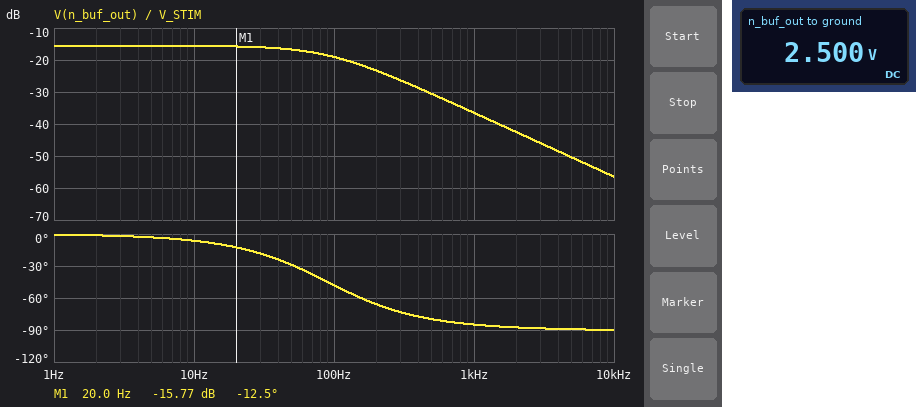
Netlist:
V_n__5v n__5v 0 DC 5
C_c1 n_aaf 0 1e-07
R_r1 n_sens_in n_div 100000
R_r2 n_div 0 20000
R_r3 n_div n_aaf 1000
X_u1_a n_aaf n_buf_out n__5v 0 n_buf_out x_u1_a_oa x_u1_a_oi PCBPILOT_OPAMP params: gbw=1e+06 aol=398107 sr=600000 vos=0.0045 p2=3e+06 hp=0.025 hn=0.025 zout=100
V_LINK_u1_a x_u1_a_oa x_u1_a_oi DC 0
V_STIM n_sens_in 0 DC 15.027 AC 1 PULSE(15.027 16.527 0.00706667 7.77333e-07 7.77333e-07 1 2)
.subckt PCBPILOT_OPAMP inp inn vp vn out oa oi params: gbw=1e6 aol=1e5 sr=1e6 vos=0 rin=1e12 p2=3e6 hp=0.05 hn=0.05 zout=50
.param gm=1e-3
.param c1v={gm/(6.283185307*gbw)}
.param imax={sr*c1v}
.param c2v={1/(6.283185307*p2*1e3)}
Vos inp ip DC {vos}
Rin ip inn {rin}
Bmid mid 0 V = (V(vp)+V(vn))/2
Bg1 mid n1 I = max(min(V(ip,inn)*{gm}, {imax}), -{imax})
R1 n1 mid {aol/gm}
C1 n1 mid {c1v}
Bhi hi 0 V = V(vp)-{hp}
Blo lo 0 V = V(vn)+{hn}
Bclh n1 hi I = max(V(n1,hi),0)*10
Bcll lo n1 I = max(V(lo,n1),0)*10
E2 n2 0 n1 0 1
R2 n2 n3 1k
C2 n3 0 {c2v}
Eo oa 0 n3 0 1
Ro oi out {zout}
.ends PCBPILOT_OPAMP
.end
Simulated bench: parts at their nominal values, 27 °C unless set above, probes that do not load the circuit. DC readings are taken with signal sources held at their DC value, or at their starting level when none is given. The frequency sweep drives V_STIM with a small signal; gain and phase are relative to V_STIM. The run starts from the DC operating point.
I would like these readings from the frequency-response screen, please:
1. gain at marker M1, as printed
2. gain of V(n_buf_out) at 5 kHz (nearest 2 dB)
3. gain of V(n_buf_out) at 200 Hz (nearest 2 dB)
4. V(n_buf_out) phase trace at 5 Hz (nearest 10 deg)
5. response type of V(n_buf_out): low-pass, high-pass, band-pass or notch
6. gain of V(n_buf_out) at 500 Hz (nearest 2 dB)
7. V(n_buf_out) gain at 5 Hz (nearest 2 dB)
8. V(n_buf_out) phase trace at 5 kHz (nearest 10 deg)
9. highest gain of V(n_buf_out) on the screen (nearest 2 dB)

-15.77 dB
-50 dB
-24 dB
0 deg
low-pass
-30 dB
-16 dB
-90 deg
-16 dB
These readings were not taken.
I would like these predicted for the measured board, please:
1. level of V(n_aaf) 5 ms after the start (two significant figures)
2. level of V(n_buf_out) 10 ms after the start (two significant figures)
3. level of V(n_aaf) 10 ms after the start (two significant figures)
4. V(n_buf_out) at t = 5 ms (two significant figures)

2.5 V
2.7 V
2.7 V
2.5 V
